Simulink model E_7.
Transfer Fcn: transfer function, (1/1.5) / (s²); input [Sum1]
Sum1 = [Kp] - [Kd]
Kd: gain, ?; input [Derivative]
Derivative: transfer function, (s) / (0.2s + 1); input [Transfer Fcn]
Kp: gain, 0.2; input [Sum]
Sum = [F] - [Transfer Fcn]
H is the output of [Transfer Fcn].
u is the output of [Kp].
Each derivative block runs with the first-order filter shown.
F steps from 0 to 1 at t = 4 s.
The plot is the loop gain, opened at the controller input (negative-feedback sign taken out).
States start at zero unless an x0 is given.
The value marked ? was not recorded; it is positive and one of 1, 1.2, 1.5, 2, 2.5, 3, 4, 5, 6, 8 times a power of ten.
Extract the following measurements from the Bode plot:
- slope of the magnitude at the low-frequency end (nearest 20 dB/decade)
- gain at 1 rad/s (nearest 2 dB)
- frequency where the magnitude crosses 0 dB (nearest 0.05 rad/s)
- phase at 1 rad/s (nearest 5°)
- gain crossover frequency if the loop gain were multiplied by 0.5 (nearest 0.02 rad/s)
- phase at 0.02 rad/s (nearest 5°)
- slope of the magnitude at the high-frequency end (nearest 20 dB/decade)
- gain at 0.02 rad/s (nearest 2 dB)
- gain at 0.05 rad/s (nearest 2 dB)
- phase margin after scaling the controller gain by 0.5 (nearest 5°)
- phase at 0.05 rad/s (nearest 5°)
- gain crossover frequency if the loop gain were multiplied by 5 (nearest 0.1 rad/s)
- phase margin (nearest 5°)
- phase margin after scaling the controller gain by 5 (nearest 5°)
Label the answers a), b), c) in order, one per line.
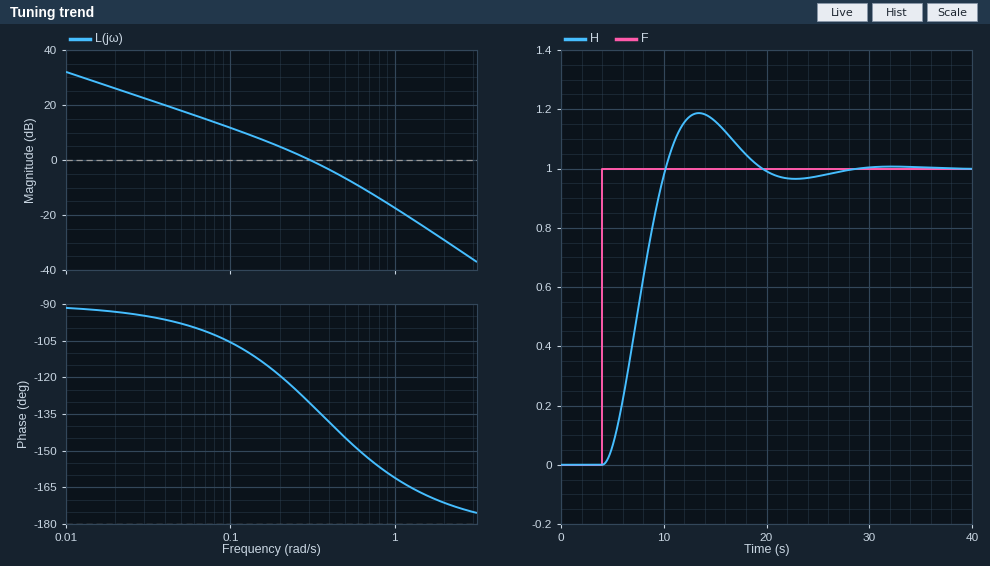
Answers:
a) -20 dB/decade
b) -18 dB
c) 0.30 rad/s
d) -160°
e) 0.18 rad/s
f) -95°
g) -40 dB/decade
h) 26 dB
i) 18 dB
j) 65°
k) -100°
l) 0.8 rad/s
m) 50°
n) 25°
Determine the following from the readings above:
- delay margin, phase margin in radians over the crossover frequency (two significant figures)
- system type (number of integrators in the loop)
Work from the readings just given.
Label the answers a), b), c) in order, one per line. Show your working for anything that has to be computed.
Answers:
a) 50 × π / 180 / 0.3 = 2.9 s
b) 1
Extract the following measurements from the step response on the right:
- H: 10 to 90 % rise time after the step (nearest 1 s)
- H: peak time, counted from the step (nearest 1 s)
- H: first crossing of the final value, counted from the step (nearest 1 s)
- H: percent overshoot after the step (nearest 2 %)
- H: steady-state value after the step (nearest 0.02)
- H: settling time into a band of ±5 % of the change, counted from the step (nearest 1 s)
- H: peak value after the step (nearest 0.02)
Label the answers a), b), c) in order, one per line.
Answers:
a) 4 s
b) 9 s
c) 6 s
d) 18 %
e) 1.00
f) 14 s
g) 1.18
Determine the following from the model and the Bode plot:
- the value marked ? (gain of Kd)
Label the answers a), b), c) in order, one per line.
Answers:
a) 0.5
